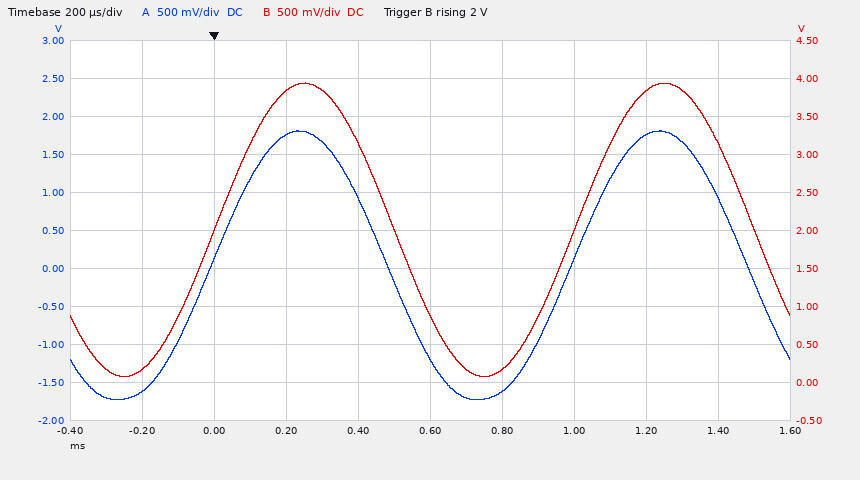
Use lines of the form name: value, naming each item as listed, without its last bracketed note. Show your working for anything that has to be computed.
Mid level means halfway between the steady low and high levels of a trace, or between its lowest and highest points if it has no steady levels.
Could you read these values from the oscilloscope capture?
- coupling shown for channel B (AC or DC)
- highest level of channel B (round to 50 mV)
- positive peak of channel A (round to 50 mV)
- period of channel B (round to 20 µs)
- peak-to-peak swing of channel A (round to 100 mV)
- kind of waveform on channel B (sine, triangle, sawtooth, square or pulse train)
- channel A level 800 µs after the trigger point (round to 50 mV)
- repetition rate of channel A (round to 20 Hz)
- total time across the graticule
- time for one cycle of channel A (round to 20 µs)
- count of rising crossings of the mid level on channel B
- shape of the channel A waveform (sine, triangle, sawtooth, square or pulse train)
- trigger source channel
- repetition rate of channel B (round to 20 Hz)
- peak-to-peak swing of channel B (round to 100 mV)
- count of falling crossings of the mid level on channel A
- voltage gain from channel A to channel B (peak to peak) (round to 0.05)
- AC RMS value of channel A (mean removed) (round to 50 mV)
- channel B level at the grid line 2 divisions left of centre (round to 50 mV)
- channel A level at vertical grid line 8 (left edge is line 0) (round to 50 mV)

coupling shown for channel B: DC
highest level of channel B: 3.95 V
positive peak of channel A: 1.80 V
period of channel B: 1.00 ms
peak-to-peak swing of channel A: 3.50 V
kind of waveform on channel B: sine
channel A level 800 µs after the trigger point: -1.60 V
repetition rate of channel A: 1 / 1.00 ms ≈ 1.00 kHz
total time across the graticule: 2 ms
time for one cycle of channel A: 1.00 ms
count of rising crossings of the mid level on channel B: 2
shape of the channel A waveform: sine
trigger source channel: channel B
repetition rate of channel B: 1 / 1.00 ms ≈ 1.00 kHz
peak-to-peak swing of channel B: 3.90 V
count of falling crossings of the mid level on channel A: 2
voltage gain from channel A to channel B (peak to peak): 3.90 V / 3.50 V ≈ 1.11, so 1.10 to the nearest 0.05
AC RMS value of channel A (mean removed): 3.50 V / (2√2) ≈ 1.24 V, so 1.25 V to the nearest 50 mV
channel B level at the grid line 2 divisions left of centre: 3.85 V
channel A level at vertical grid line 8 (left edge is line 0): 1.75 V
